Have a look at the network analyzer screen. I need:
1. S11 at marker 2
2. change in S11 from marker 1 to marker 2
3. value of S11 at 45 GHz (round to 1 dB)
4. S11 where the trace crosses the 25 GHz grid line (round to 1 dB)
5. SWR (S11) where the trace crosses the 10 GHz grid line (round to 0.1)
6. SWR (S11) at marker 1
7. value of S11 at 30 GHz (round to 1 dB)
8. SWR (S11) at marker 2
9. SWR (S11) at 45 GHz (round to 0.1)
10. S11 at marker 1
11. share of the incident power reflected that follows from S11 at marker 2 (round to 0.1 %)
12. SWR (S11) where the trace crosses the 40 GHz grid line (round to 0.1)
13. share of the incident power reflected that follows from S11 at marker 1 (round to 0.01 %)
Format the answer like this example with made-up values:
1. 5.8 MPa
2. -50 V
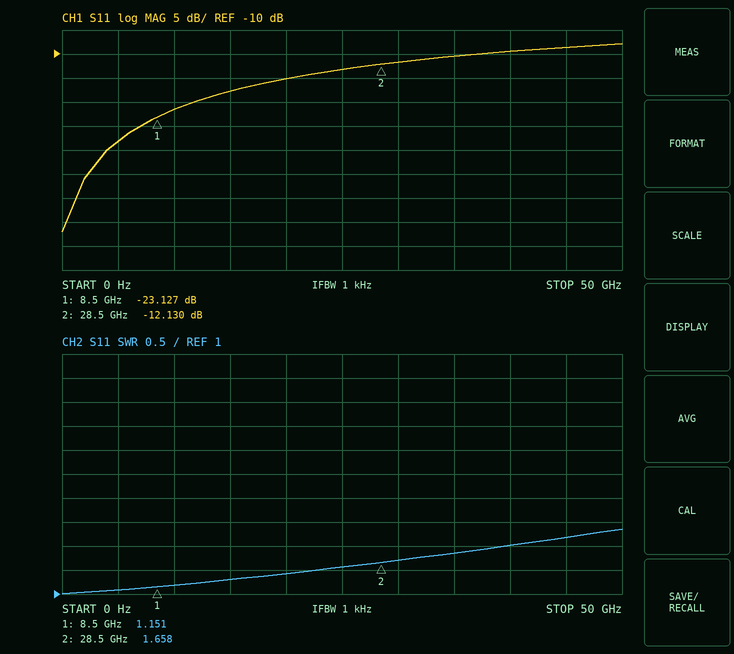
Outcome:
1. -12.130 dB
2. 10.997 dB
3. -9 dB
4. -13 dB
5. 1.2
6. 1.151
7. -12 dB
8. 1.658
9. 2.2
10. -23.127 dB
11. 6.1 %
12. 2.0
13. 0.49 %
